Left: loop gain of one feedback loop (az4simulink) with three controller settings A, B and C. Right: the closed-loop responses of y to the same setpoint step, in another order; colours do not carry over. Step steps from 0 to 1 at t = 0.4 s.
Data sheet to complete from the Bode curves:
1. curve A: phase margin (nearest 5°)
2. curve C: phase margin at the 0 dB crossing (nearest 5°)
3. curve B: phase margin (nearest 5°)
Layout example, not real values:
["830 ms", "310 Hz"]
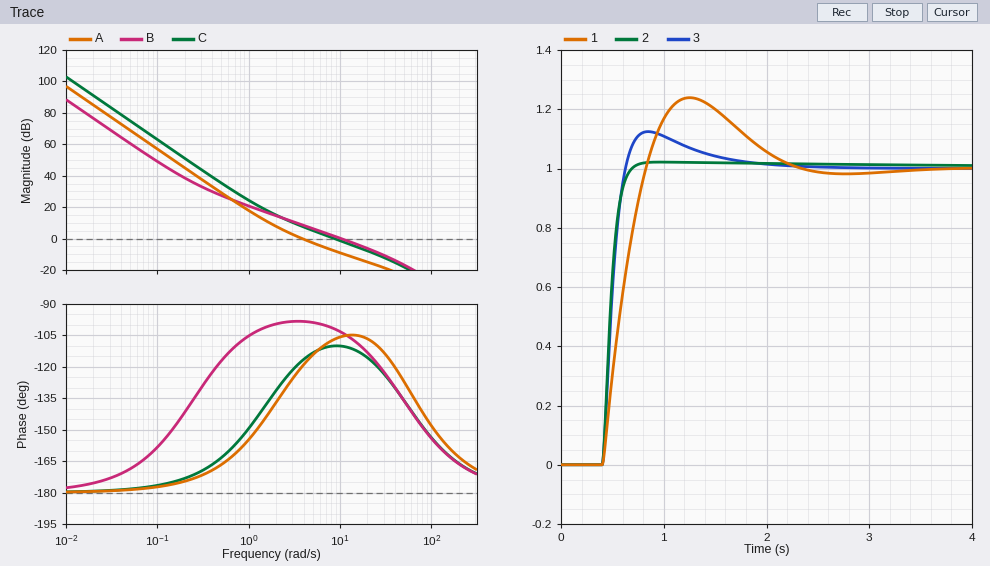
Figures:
["60°", "70°", "75°"]
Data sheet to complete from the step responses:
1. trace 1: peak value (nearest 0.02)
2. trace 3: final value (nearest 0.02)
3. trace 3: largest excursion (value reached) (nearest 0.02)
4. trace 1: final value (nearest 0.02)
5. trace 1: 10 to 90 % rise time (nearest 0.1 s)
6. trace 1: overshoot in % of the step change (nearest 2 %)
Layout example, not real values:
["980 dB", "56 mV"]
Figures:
["1.24", "1.00", "1.12", "1.00", "0.3 s", "24 %"]
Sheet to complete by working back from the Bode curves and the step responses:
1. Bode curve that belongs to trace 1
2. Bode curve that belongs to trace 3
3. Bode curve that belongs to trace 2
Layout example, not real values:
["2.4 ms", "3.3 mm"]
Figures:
["A", "C", "B"]
